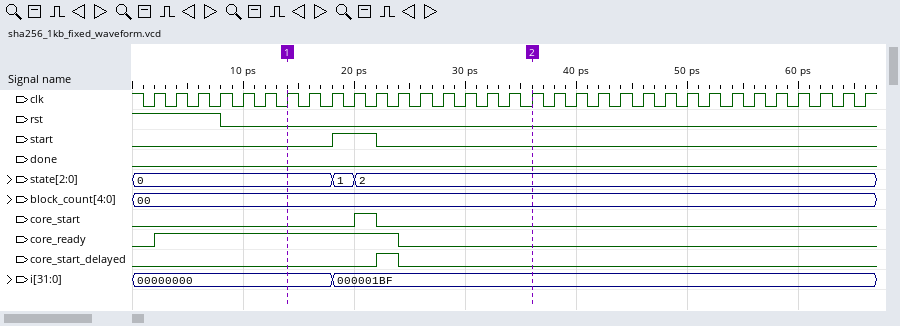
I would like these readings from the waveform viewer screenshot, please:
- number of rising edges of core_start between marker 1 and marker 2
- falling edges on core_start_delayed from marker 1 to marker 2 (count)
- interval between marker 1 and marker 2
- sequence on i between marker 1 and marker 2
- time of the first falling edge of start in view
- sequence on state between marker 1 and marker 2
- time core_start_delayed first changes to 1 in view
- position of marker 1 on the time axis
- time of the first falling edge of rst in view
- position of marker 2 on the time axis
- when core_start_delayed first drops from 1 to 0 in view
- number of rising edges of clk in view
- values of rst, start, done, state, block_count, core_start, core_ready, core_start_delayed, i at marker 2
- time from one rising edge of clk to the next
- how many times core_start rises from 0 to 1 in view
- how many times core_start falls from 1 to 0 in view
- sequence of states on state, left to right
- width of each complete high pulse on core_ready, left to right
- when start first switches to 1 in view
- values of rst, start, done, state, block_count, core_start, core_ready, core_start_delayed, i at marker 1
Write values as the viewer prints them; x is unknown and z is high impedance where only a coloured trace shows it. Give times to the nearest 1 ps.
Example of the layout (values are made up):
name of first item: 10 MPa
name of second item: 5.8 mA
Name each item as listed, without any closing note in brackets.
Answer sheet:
number of rising edges of core_start between marker 1 and marker 2: 1
falling edges on core_start_delayed from marker 1 to marker 2: 1
interval between marker 1 and marker 2: 22 ps
sequence on i between marker 1 and marker 2: 00000000, 000001BF
time of the first falling edge of start in view: 22 ps
sequence on state between marker 1 and marker 2: 0, 1, 2
time core_start_delayed first changes to 1 in view: 22 ps
position of marker 1 on the time axis: 14 ps
time of the first falling edge of rst in view: 8 ps
position of marker 2 on the time axis: 36 ps
when core_start_delayed first drops from 1 to 0 in view: 24 ps
number of rising edges of clk in view: 33
values of rst, start, done, state, block_count, core_start, core_ready, core_start_delayed, i at marker 2: rst=0, start=0, done=0, state=2, block_count=00, core_start=0, core_ready=0, core_start_delayed=0, i=000001BF
time from one rising edge of clk to the next: 2 ps
how many times core_start rises from 0 to 1 in view: 1
how many times core_start falls from 1 to 0 in view: 1
sequence of states on state, left to right: 0, 1, 2
width of each complete high pulse on core_ready, left to right: 22 ps
when start first switches to 1 in view: 18 ps
values of rst, start, done, state, block_count, core_start, core_ready, core_start_delayed, i at marker 1: rst=0, start=0, done=0, state=0, block_count=00, core_start=0, core_ready=1, core_start_delayed=0, i=00000000
